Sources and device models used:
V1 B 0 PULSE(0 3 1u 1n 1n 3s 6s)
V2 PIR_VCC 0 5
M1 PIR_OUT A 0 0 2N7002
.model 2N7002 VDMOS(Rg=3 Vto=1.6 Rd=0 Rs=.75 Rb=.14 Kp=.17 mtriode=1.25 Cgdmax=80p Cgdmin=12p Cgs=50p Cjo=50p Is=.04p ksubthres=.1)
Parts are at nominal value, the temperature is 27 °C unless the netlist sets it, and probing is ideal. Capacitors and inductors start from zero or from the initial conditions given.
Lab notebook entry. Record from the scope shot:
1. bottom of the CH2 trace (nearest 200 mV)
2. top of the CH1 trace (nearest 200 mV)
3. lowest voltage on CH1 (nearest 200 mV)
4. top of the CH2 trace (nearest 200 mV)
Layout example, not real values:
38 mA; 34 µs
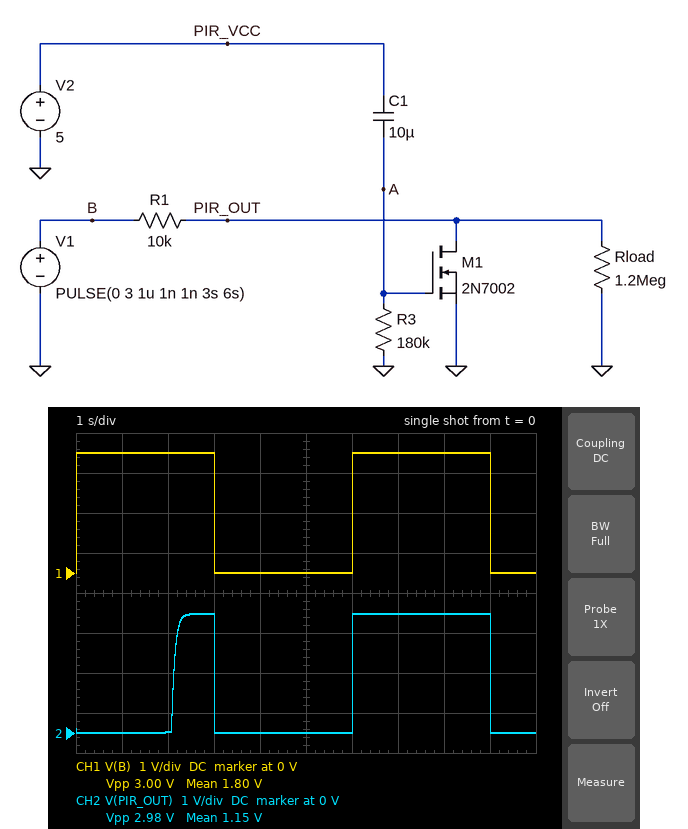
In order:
0 V; 3.0 V; 0 V; 3.0 V
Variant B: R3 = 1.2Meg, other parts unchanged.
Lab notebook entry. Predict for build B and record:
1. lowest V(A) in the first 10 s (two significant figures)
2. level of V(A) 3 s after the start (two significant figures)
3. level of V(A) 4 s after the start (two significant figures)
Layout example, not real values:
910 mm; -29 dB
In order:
2.2 V; 3.9 V; 3.6 V
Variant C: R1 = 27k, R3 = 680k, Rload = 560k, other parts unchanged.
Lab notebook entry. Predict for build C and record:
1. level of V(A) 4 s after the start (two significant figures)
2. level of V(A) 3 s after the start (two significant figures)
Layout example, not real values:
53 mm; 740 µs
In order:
2.8 V; 3.2 V
